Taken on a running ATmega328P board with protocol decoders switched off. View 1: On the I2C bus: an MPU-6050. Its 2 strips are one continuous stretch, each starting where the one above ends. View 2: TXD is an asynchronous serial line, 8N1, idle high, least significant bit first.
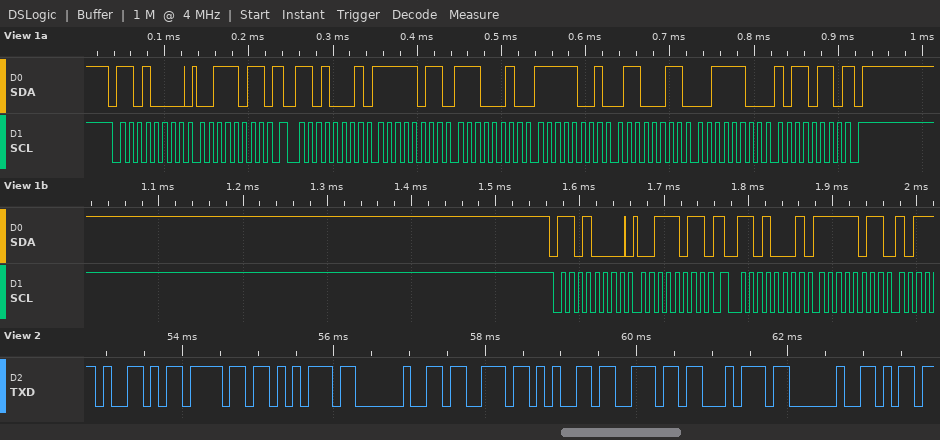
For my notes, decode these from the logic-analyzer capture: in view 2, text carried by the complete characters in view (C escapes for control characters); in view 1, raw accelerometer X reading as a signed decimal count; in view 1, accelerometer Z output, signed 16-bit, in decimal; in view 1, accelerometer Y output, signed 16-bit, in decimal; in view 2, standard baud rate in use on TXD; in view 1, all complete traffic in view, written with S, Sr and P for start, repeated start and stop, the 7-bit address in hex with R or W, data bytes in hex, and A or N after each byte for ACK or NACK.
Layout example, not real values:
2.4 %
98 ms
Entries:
"You sent "
-1054
15542
-1693
9600 baud
S 68W A 3B A Sr 68R A FB A E2 A F9 A 63 A 3C A B6 N P S 68W A 3B A Sr 68R A FB A
